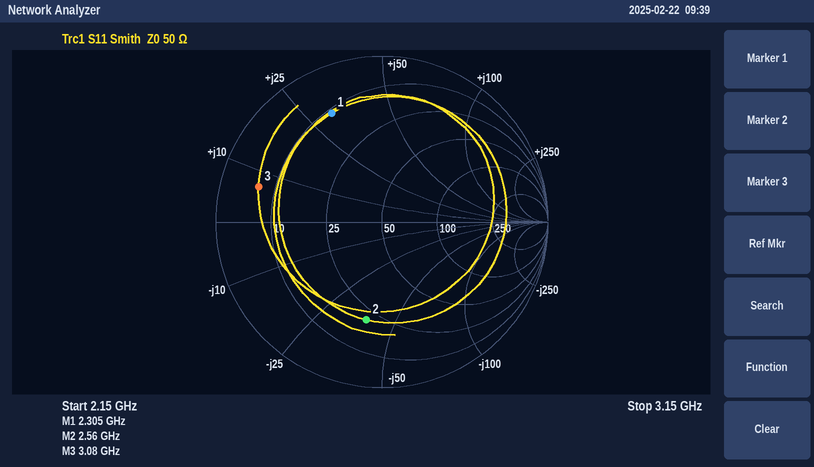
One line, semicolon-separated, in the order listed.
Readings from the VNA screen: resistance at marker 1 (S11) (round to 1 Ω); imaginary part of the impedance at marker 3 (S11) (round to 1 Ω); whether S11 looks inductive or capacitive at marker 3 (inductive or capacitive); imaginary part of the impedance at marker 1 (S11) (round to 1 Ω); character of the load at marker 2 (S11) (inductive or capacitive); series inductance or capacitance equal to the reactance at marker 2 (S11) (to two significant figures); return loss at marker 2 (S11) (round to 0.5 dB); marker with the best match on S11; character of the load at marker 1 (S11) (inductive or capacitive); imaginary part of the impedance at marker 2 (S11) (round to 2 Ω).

11 Ω; +7 Ω; inductive; +31 Ω; capacitive; 1.6 pF; 4.5 dB; marker 2; inductive; -38 Ω
